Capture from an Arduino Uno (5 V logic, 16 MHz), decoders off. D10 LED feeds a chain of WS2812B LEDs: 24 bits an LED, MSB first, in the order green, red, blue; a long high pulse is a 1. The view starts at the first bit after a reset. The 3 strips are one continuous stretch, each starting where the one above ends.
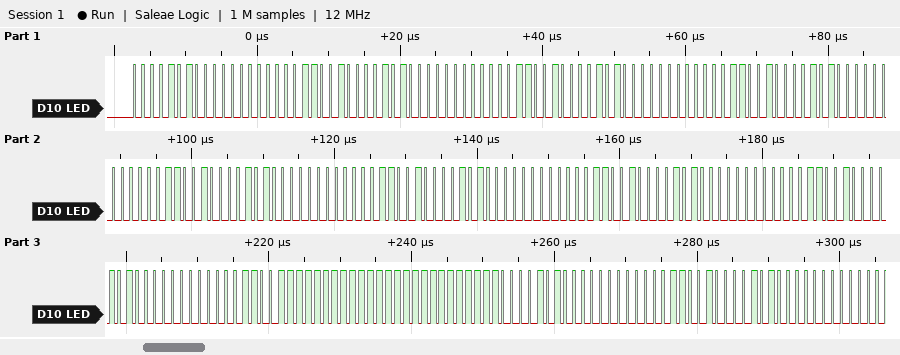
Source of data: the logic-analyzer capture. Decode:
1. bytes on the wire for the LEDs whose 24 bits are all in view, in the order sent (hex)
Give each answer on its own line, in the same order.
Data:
0A 00 19 0A 00 19 0A 00 19 0A 00 19 0A 00 19 0A 00 19 0A 00 19 0A 00 19 FF FF FF 0A 00 19
